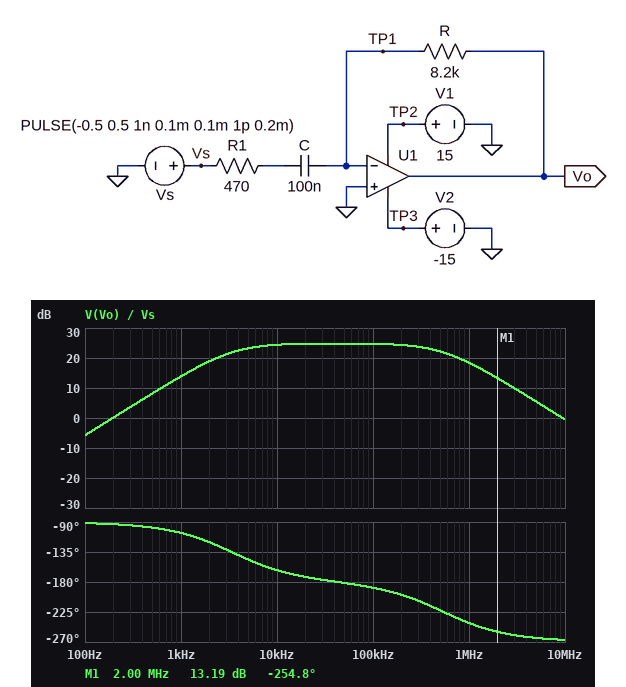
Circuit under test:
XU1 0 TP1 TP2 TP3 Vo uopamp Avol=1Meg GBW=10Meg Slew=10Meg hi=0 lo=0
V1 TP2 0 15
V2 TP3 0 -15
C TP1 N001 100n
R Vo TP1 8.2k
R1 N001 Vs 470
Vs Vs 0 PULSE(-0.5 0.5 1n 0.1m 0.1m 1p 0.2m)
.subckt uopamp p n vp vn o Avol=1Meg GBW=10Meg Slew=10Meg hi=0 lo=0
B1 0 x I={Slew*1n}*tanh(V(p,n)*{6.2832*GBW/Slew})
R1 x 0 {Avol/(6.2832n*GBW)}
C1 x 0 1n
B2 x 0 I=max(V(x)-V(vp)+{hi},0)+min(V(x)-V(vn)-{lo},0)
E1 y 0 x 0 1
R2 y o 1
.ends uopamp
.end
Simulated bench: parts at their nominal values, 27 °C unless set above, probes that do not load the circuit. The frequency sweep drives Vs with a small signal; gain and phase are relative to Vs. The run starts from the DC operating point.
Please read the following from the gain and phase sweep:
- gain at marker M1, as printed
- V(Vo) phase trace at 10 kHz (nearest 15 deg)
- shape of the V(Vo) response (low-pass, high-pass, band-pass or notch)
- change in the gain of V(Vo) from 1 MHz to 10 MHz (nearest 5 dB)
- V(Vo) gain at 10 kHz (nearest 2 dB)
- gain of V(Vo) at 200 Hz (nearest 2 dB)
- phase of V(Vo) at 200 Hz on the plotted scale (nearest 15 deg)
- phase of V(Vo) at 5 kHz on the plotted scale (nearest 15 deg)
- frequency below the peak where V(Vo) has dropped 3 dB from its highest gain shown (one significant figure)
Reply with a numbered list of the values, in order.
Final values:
1. 13.19 dB
2. -165 deg
3. band-pass
4. -20 dB
5. 24 dB
6. 0 dB
7. -90 deg
8. -150 deg
9. 3 kHz
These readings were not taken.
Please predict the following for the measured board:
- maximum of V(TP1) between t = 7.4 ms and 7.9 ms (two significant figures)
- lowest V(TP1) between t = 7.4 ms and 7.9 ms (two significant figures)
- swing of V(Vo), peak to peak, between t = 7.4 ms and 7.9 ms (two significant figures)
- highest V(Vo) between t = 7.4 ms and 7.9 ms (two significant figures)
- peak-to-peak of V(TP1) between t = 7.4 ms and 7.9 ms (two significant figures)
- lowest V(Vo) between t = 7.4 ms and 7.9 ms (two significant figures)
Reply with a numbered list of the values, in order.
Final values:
1. 4.9 mV
2. -4.9 mV
3. 13 V
4. 6.5 V
5. 9.8 mV
6. -6.5 V
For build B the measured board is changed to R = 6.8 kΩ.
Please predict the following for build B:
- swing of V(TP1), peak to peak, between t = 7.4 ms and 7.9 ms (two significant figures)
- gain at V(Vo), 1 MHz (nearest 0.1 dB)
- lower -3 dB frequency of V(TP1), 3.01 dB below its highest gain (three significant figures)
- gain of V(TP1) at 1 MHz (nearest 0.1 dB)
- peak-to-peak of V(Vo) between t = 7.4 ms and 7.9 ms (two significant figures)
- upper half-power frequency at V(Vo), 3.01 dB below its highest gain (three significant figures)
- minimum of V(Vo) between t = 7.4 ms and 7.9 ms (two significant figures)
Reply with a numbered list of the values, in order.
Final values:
1. 8.2 mV
2. 17.9 dB
3. 643 kHz
4. -2.1 dB
5. 11 V
6. 650 kHz
7. -5.4 V
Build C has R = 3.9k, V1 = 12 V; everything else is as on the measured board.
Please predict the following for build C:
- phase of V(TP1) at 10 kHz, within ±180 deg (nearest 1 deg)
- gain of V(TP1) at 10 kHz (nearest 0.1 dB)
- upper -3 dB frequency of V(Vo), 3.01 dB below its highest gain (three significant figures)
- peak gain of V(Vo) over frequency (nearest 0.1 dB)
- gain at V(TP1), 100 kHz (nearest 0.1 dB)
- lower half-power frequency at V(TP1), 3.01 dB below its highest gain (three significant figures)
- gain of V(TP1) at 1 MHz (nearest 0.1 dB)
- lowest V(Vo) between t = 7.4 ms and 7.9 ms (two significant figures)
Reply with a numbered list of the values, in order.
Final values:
1. 108 deg
2. -42.1 dB
3. 1.08 MHz
4. 18.4 dB
5. -21.6 dB
6. 1.07 MHz
7. -4.3 dB
8. -3.1 V
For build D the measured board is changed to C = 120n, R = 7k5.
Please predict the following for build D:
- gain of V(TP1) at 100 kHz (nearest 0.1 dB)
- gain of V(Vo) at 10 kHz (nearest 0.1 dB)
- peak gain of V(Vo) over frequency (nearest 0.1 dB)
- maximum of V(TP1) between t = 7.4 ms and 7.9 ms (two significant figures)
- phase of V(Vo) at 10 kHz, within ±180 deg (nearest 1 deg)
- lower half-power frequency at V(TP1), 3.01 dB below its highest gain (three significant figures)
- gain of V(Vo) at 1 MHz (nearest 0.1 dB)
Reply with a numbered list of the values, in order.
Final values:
1. -16.0 dB
2. 23.8 dB
3. 24.1 dB
4. 4.3 mV
5. -165 deg
6. 587 kHz
7. 18.2 dB
